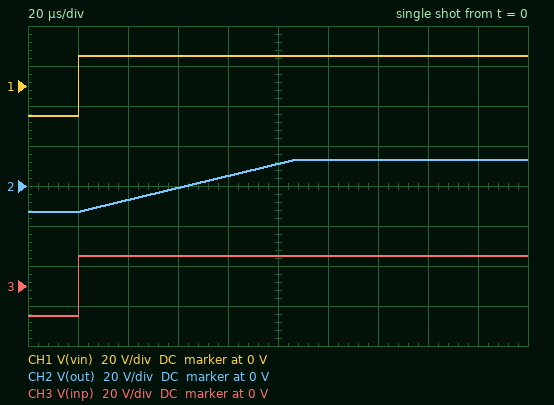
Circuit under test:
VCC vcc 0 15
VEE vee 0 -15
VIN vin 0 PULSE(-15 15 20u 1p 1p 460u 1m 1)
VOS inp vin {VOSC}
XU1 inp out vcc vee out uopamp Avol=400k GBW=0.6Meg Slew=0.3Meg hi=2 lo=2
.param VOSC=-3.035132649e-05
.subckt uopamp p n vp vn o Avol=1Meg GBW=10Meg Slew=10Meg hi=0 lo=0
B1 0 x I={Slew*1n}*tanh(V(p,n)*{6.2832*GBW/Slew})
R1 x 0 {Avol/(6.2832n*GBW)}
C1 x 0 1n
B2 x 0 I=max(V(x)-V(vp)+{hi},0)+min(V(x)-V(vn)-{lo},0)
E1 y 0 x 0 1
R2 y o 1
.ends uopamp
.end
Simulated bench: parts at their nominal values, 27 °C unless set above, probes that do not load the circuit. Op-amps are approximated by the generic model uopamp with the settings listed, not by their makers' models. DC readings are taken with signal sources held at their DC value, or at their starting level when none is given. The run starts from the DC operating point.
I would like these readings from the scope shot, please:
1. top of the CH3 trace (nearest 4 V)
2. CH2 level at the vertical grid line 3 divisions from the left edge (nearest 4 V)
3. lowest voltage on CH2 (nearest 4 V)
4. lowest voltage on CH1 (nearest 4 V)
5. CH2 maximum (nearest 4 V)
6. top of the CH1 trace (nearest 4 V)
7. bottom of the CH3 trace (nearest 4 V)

16 V
0 V
-12 V
-16 V
12 V
16 V
-16 V
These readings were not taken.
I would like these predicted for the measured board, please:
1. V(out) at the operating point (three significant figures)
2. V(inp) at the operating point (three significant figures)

-13.0 V
-15.0 V
